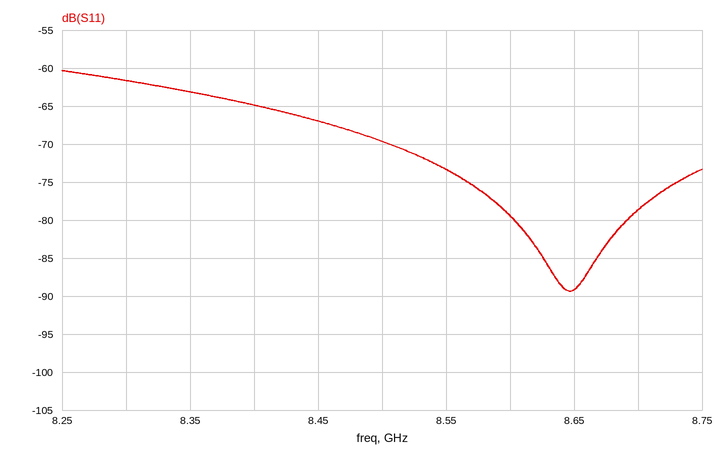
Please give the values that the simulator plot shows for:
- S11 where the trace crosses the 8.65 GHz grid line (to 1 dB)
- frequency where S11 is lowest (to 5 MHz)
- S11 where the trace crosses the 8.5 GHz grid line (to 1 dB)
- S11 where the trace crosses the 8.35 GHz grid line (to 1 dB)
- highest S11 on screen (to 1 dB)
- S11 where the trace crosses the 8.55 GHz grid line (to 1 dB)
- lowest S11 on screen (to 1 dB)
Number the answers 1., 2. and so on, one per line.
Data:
1. -89 dB
2. 8.645 GHz
3. -70 dB
4. -63 dB
5. -60 dB
6. -73 dB
7. -89 dB
